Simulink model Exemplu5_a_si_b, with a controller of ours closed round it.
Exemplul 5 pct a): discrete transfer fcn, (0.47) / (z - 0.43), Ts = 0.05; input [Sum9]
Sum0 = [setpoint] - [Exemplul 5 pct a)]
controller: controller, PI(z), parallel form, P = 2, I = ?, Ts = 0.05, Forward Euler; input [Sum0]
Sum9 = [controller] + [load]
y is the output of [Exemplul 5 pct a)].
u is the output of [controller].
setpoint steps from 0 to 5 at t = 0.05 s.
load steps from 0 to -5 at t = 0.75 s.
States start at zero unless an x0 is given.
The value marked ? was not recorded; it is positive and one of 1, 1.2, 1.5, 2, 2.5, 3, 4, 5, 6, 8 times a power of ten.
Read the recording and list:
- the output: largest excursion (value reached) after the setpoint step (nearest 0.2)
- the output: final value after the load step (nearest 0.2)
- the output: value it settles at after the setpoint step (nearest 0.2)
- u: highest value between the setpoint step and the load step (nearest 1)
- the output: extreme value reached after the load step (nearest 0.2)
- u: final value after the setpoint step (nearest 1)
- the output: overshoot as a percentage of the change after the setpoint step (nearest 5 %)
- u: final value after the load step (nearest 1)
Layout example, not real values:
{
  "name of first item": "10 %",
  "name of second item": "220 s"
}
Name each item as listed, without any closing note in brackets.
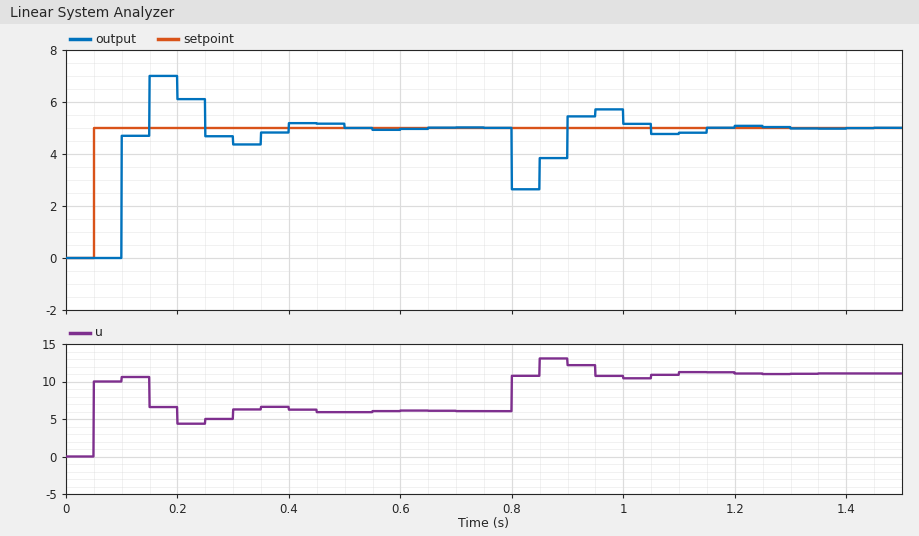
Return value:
{
  "the output: largest excursion (value reached) after the setpoint step": "7.0",
  "the output: final value after the load step": "5.0",
  "the output: value it settles at after the setpoint step": "5.0",
  "u: highest value between the setpoint step and the load step": "11",
  "the output: extreme value reached after the load step": "2.6",
  "u: final value after the setpoint step": "6",
  "the output: overshoot as a percentage of the change after the setpoint step": "40 %",
  "u: final value after the load step": "11"
}
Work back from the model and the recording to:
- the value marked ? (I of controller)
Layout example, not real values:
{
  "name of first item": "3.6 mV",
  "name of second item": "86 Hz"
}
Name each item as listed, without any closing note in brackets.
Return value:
{
  "the value marked ?": "40"
}
